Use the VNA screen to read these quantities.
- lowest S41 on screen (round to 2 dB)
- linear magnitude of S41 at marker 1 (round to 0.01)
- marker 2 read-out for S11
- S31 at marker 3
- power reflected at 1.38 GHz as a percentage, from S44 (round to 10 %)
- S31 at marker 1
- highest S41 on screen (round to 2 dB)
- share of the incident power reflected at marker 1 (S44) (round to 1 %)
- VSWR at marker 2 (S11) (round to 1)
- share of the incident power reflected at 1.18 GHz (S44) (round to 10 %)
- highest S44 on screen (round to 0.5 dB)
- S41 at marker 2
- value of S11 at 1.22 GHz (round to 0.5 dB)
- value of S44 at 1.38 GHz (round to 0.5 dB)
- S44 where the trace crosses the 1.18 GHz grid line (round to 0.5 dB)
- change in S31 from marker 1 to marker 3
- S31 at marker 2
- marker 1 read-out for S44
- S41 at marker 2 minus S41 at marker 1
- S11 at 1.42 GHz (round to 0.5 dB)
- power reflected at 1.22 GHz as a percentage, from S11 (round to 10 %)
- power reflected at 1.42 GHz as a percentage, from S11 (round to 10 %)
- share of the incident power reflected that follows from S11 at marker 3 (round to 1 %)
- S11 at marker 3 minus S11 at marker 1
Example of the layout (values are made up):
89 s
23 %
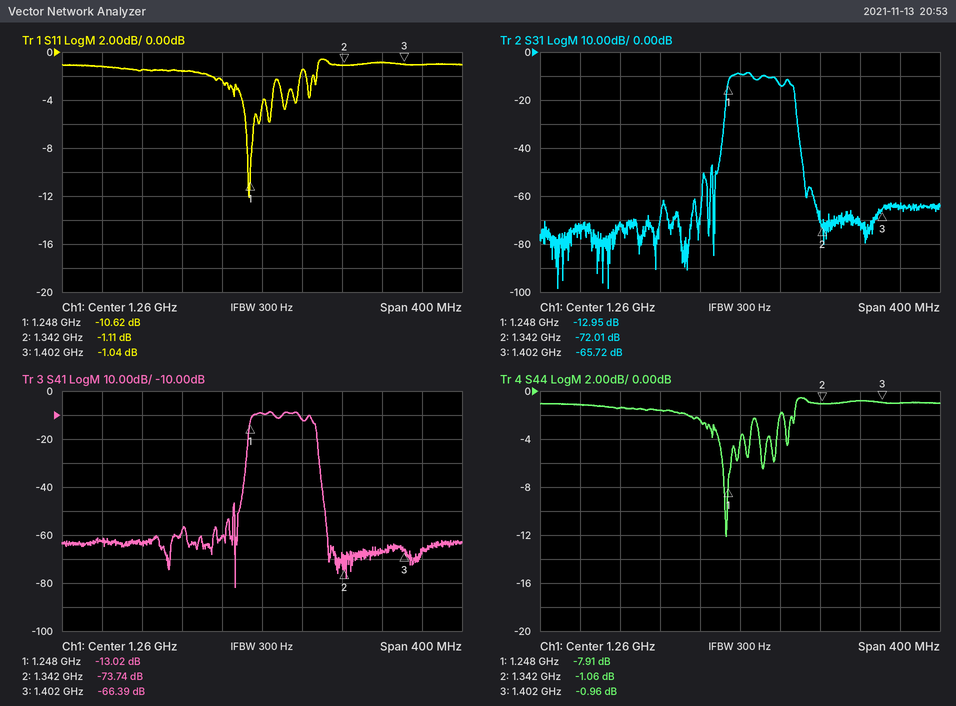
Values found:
-82 dB
0.22
-1.11 dB
-65.72 dB
80 %
-12.95 dB
-8 dB
16 %
16
70 %
-0.5 dB
-73.74 dB
-2.5 dB
-1.0 dB
-1.5 dB
-52.77 dB
-72.01 dB
-7.91 dB
-60.72 dB
-1.0 dB
60 %
80 %
79 %
9.58 dB
